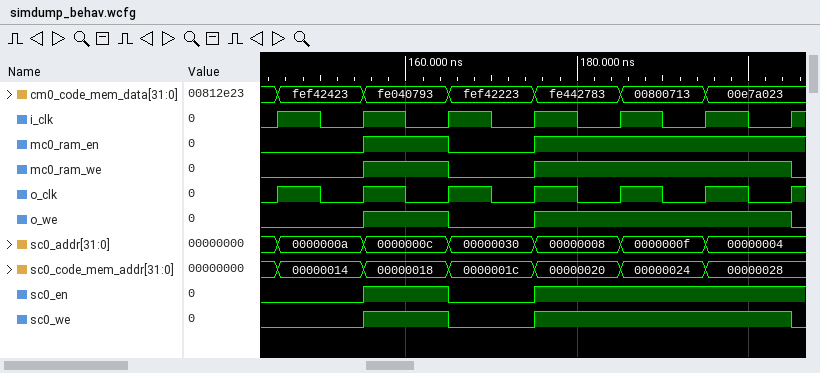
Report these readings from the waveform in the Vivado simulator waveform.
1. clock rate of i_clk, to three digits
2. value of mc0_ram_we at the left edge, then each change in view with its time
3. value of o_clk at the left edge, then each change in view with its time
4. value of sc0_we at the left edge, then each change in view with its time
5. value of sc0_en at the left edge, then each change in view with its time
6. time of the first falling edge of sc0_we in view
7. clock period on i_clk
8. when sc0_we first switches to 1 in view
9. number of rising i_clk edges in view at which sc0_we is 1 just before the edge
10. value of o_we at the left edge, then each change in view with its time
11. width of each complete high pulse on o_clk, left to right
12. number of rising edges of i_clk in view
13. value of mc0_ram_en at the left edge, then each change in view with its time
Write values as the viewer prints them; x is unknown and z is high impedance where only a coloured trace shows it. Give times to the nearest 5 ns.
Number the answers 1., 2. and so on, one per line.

1. 100 MHz
2. 0, 1 at 155 ns, 0 at 165 ns, 1 at 175 ns, 0 at 205 ns
3. 0, 1 at 145 ns, 0 at 150 ns, 1 at 155 ns, 0 at 160 ns, 1 at 165 ns, 0 at 170 ns, 1 at 175 ns, 0 at 180 ns, 1 at 185 ns, 0 at 190 ns, 1 at 195 ns, 0 at 200 ns, 1 at 205 ns
4. 0, 1 at 155 ns, 0 at 165 ns, 1 at 175 ns, 0 at 205 ns
5. 0, 1 at 155 ns, 0 at 165 ns, 1 at 175 ns
6. 165 ns
7. 10 ns
8. 155 ns
9. 4
10. 0, 1 at 155 ns, 0 at 165 ns, 1 at 175 ns, 0 at 205 ns
11. 5 ns, 5 ns, 5 ns, 5 ns, 5 ns, 5 ns
12. 7
13. 0, 1 at 155 ns, 0 at 165 ns, 1 at 175 ns
